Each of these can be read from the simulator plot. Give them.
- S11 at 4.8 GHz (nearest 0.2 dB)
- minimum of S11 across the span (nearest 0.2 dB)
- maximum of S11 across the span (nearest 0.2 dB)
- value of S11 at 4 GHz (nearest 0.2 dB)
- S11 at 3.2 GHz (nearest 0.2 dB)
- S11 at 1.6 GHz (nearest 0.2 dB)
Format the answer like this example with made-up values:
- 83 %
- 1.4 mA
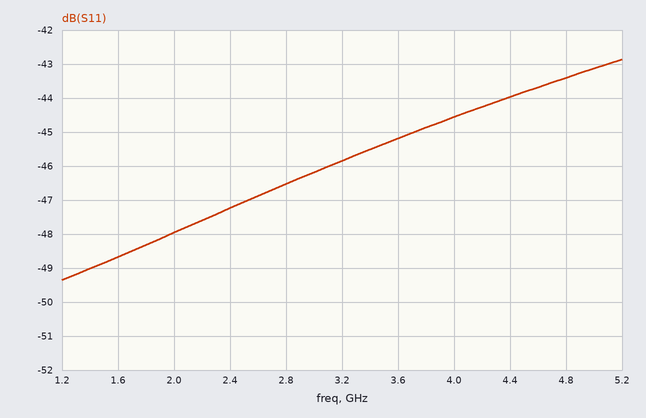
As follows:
- -43.4 dB
- -49.4 dB
- -42.8 dB
- -44.6 dB
- -45.8 dB
- -48.6 dB
